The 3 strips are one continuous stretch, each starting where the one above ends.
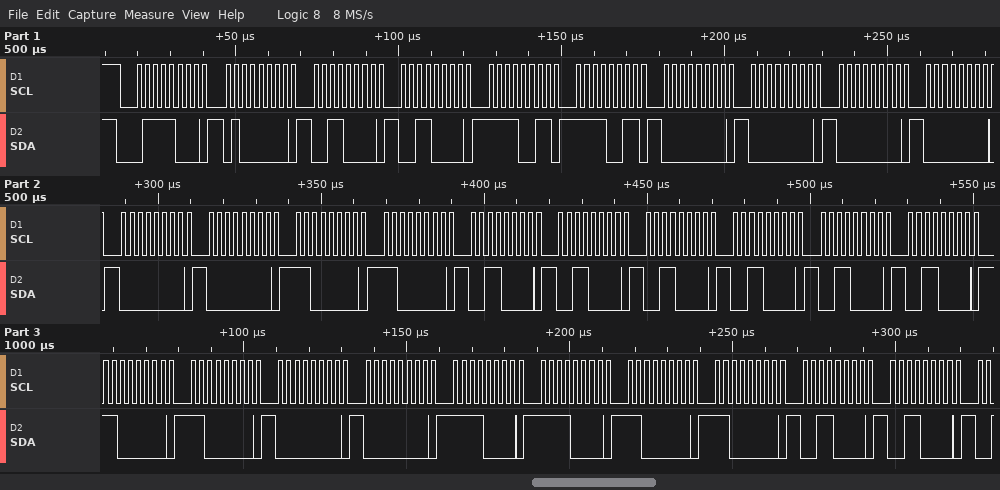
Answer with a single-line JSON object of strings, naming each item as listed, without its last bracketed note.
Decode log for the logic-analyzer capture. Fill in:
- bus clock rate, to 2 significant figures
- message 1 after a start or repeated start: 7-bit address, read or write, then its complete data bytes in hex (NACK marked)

{"bus clock rate, to 2 significant figures": "400 kHz", "message 1 after a start or repeated start: 7-bit address, read or write, then its complete data bytes in hex": "0x3C write: 40 30 30 F3 F3 00 00 00 00 00 00 C0 C0 30 30 30 30 30 30 C0 C0 00 00 F0 F0 C0 C0 30 30"}
